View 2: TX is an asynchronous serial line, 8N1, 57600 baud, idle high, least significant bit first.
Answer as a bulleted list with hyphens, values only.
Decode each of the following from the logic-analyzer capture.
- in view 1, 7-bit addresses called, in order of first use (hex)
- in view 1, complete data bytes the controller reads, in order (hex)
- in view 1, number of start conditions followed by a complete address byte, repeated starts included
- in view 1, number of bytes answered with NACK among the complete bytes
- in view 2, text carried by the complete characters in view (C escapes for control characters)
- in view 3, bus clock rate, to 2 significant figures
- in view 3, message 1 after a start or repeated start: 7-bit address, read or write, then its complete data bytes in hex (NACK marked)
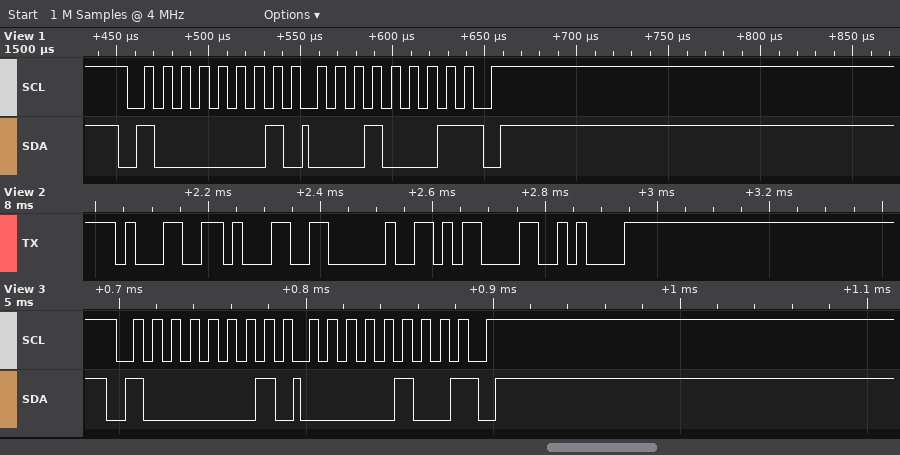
- 0x40
- 11
- 1
- 1
- "11 \r\n"
- 100 kHz
- 0x40 read: 04 NACK
